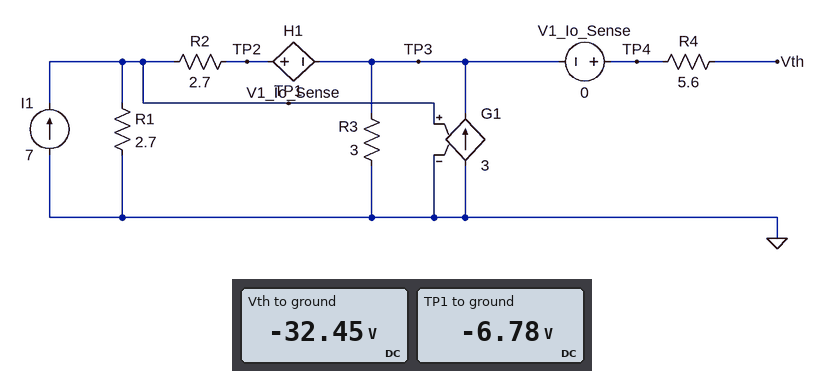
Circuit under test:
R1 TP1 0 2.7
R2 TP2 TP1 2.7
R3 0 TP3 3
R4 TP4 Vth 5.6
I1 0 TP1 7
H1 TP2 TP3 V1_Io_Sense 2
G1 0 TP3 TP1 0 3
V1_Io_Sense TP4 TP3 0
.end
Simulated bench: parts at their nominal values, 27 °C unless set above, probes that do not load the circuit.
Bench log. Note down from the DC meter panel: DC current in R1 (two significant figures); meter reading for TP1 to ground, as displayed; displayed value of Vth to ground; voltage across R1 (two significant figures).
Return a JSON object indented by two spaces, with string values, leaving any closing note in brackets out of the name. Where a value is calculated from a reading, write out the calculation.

{
  "DC current in R1": "(0 V - (-6.78 V)) / 2.7 Ω = 2.5 A",
  "meter reading for TP1 to ground, as displayed": "-6.78 V",
  "displayed value of Vth to ground": "-32.45 V",
  "voltage across R1": "0 V - (-6.78 V) = 6.8 V"
}
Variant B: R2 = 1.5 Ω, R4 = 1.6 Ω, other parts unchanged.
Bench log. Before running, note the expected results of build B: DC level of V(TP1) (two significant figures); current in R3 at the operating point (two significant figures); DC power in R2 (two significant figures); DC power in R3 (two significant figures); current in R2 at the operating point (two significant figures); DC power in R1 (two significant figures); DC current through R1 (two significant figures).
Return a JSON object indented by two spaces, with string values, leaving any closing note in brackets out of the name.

{
  "DC level of V(TP1)": "-5.0 V",
  "current in R3 at the operating point": "6.1 A",
  "DC power in R2": "120 W",
  "DC power in R3": "110 W",
  "current in R2 at the operating point": "8.8 A",
  "DC power in R1": "9.2 W",
  "DC current through R1": "1.8 A"
}
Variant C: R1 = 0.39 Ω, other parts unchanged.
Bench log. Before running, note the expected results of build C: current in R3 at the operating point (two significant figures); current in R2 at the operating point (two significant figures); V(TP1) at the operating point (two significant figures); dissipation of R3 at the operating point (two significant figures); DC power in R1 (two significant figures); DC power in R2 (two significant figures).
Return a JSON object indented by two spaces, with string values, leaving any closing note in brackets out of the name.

{
  "current in R3 at the operating point": "9.6 A",
  "current in R2 at the operating point": "8.5 A",
  "V(TP1) at the operating point": "6.0 V",
  "dissipation of R3 at the operating point": "280 W",
  "DC power in R1": "93 W",
  "DC power in R2": "190 W"
}
